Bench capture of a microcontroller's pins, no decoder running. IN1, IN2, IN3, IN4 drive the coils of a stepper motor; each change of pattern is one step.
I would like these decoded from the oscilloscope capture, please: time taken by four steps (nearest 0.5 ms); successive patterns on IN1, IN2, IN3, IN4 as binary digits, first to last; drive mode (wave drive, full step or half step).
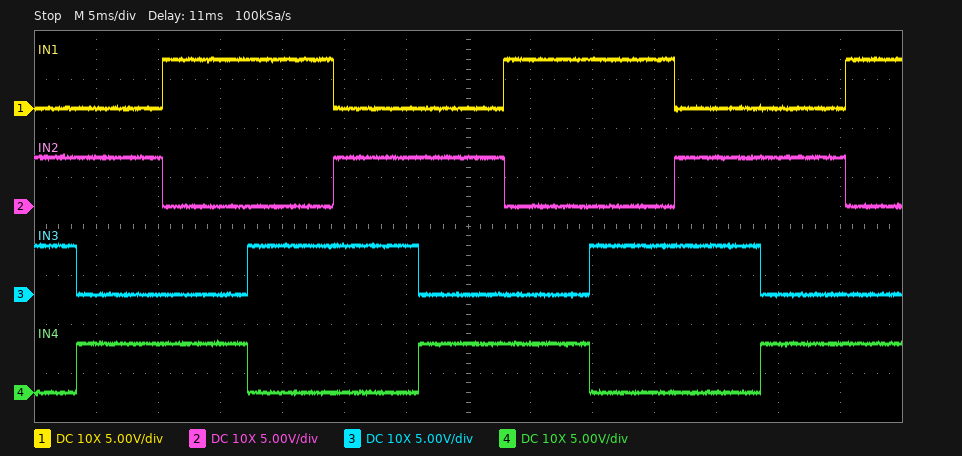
27.5 ms
0110 0101 1001 1010 0110 0101 1001 1010 0110 0101 1001
full step
